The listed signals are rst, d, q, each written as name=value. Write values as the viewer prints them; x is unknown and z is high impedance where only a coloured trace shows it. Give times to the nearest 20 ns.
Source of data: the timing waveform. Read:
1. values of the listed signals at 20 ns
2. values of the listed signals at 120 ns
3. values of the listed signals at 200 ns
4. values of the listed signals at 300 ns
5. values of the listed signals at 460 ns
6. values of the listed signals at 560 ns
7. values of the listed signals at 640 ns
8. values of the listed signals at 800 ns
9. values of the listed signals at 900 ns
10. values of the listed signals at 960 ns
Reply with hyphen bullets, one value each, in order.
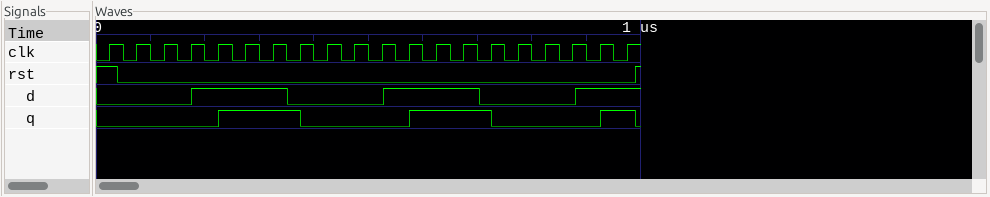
- rst=1, d=0, q=0
- rst=0, d=0, q=0
- rst=0, d=1, q=0
- rst=0, d=1, q=1
- rst=0, d=0, q=0
- rst=0, d=1, q=0
- rst=0, d=1, q=1
- rst=0, d=0, q=0
- rst=0, d=1, q=0
- rst=0, d=1, q=1
